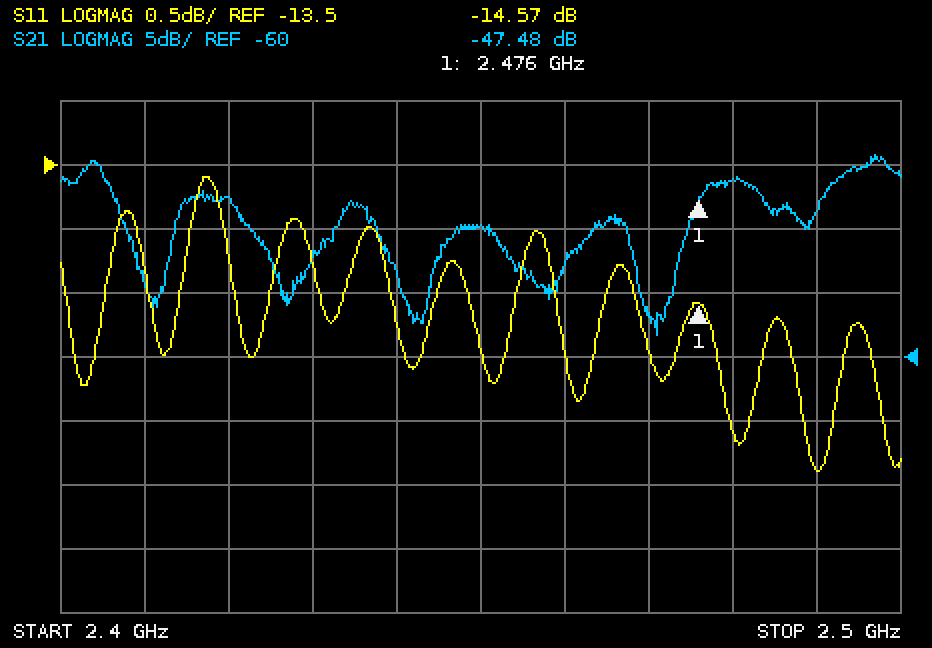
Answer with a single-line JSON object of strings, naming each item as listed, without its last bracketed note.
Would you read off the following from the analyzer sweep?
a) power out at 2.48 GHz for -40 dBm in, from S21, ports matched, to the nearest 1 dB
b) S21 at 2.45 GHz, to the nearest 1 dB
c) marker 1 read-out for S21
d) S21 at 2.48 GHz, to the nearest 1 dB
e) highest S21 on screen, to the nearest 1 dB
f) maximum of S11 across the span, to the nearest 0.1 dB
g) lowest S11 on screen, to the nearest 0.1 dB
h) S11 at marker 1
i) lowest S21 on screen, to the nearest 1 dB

{"power out at 2.48 GHz for -40 dBm in, from S21, ports matched, to the nearest 1 dB": "-86 dBm", "S21 at 2.45 GHz, to the nearest 1 dB": "-50 dB", "marker 1 read-out for S21": "-47.48 dB", "S21 at 2.48 GHz, to the nearest 1 dB": "-46 dB", "highest S21 on screen, to the nearest 1 dB": "-44 dB", "maximum of S11 across the span, to the nearest 0.1 dB": "-13.6 dB", "lowest S11 on screen, to the nearest 0.1 dB": "-15.9 dB", "S11 at marker 1": "-14.57 dB", "lowest S21 on screen, to the nearest 1 dB": "-58 dB"}
